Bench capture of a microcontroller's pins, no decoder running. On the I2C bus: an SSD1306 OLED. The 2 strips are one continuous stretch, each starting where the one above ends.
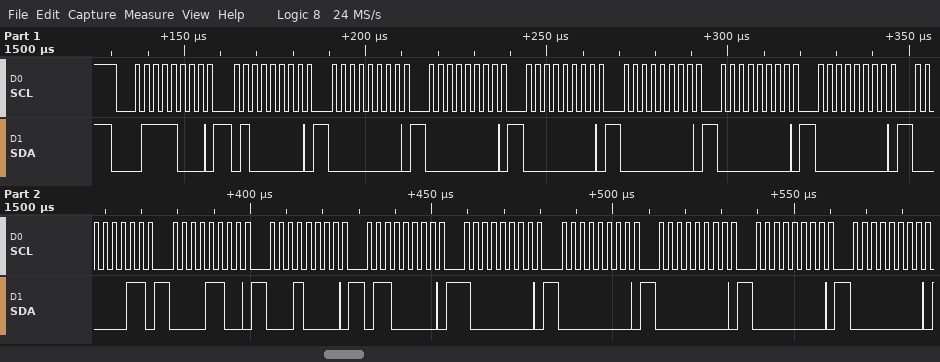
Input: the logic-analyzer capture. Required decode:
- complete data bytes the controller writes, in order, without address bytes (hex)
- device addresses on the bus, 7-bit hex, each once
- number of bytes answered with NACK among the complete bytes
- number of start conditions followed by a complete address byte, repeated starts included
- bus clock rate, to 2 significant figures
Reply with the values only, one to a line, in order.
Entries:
40 00 00 00 00 00 00 03 0C 10 60 80 00 00 00 00
0x3C
0
1
400 kHz
